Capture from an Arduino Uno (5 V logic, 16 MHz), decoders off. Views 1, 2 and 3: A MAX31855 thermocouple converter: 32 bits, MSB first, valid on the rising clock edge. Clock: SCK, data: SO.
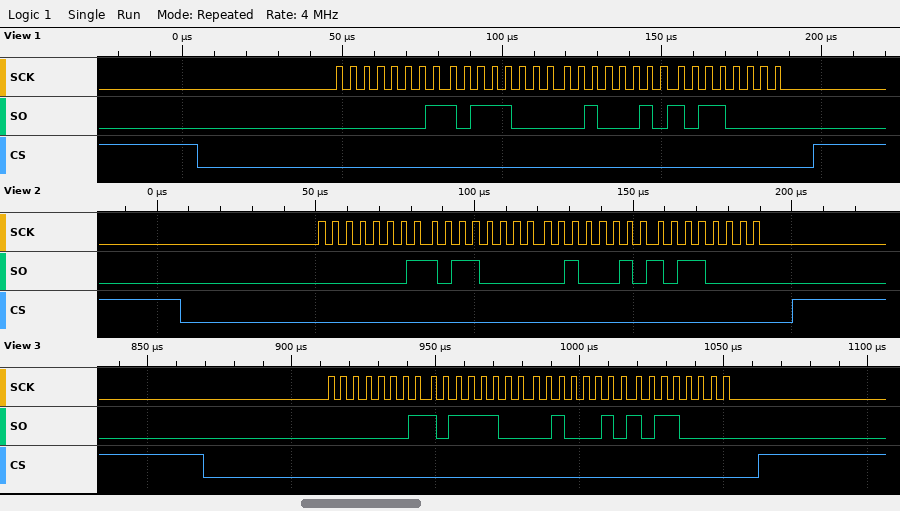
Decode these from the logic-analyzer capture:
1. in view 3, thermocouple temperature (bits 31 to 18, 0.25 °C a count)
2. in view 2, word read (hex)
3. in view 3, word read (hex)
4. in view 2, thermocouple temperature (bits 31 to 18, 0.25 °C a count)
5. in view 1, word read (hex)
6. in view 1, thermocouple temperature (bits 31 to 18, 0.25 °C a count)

27.75 °C
0x01B022B0
0x01BC22B0
27.00 °C
0x01B822B0
27.50 °C
